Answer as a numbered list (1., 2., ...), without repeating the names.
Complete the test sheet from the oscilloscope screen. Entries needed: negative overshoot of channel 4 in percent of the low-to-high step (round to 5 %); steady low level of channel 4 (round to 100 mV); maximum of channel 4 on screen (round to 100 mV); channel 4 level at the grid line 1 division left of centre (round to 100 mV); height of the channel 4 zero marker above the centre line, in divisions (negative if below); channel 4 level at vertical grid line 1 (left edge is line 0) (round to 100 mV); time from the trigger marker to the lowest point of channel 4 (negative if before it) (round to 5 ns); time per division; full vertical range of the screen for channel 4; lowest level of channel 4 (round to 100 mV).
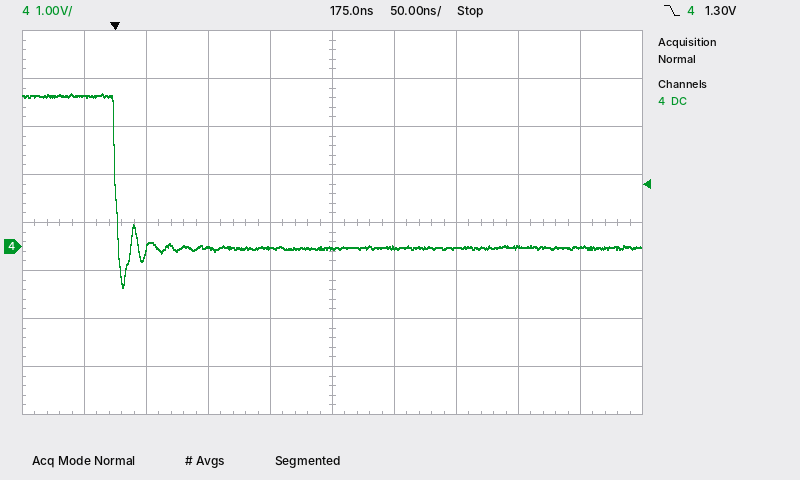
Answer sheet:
1. 25 %
2. 0.0 V
3. 3.2 V
4. 0.0 V
5. -0.5 div
6. 3.1 V
7. +5 ns
8. 50 ns
9. 8 V
10. -900 mV
